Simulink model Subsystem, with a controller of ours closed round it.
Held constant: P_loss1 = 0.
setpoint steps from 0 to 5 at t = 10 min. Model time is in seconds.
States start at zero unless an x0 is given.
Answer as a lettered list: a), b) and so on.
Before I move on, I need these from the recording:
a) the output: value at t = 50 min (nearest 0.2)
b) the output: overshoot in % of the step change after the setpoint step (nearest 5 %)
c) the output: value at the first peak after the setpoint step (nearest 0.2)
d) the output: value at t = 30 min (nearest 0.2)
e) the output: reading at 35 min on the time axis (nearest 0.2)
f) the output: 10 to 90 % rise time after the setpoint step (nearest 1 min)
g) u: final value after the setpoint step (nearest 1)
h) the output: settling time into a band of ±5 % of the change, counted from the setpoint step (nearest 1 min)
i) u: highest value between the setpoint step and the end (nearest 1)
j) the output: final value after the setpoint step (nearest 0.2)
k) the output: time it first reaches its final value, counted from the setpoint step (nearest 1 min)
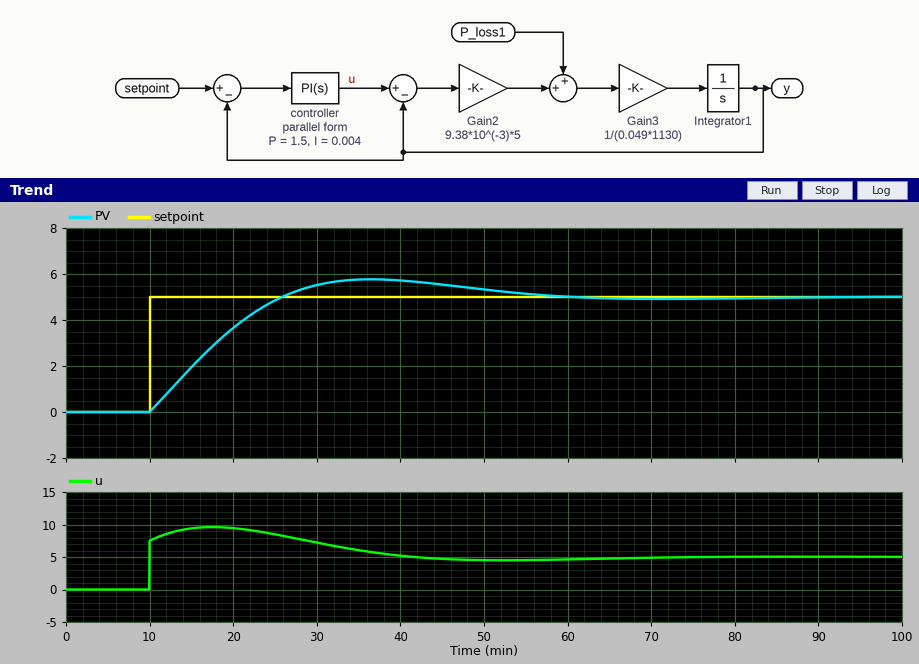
a) 5.4
b) 15 %
c) 5.8
d) 5.6
e) 5.8
f) 12 min
g) 5
h) 42 min
i) 10
j) 5.0
k) 16 min
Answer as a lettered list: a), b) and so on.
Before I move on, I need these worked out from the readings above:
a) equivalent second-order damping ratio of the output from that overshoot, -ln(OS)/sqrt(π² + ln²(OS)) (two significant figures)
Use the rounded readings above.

a) 0.52
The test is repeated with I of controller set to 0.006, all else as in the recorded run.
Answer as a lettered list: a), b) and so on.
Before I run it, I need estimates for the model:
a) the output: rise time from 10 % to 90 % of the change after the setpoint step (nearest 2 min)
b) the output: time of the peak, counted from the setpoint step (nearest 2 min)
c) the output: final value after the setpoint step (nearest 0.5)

a) 10 min
b) 22 min
c) 5.0
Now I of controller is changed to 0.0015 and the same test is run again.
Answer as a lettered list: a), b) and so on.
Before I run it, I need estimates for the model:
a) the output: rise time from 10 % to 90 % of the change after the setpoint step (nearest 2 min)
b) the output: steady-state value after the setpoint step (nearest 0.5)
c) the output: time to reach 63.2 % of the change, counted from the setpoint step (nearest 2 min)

a) 24 min
b) 5.0
c) 12 min
